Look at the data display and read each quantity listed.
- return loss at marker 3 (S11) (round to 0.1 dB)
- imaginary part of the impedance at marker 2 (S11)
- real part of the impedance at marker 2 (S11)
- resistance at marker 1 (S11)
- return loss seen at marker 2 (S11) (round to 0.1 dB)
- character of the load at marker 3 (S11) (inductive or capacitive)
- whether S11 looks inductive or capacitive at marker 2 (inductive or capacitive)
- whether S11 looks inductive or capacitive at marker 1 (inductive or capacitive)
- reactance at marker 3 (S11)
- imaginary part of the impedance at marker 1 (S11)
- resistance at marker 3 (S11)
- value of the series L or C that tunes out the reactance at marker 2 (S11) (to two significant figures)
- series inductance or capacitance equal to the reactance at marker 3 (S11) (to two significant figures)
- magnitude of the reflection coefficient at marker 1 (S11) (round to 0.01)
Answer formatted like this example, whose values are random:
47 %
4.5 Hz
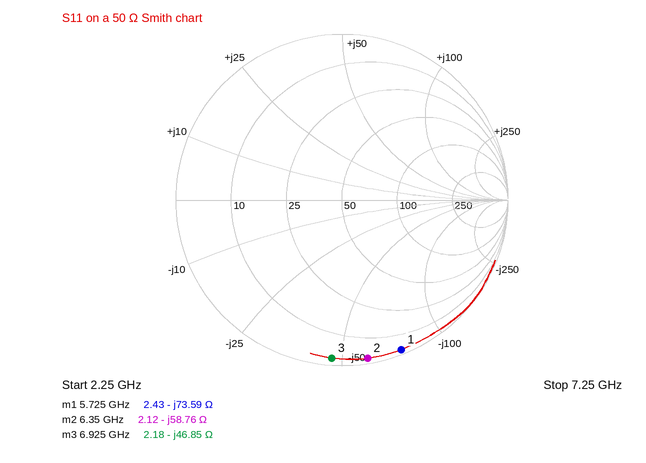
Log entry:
0.4 dB
-58.76 Ω
2.12 Ω
2.43 Ω
0.3 dB
capacitive
capacitive
capacitive
-46.85 Ω
-73.59 Ω
2.18 Ω
1.5 nH
490 fF
0.97
